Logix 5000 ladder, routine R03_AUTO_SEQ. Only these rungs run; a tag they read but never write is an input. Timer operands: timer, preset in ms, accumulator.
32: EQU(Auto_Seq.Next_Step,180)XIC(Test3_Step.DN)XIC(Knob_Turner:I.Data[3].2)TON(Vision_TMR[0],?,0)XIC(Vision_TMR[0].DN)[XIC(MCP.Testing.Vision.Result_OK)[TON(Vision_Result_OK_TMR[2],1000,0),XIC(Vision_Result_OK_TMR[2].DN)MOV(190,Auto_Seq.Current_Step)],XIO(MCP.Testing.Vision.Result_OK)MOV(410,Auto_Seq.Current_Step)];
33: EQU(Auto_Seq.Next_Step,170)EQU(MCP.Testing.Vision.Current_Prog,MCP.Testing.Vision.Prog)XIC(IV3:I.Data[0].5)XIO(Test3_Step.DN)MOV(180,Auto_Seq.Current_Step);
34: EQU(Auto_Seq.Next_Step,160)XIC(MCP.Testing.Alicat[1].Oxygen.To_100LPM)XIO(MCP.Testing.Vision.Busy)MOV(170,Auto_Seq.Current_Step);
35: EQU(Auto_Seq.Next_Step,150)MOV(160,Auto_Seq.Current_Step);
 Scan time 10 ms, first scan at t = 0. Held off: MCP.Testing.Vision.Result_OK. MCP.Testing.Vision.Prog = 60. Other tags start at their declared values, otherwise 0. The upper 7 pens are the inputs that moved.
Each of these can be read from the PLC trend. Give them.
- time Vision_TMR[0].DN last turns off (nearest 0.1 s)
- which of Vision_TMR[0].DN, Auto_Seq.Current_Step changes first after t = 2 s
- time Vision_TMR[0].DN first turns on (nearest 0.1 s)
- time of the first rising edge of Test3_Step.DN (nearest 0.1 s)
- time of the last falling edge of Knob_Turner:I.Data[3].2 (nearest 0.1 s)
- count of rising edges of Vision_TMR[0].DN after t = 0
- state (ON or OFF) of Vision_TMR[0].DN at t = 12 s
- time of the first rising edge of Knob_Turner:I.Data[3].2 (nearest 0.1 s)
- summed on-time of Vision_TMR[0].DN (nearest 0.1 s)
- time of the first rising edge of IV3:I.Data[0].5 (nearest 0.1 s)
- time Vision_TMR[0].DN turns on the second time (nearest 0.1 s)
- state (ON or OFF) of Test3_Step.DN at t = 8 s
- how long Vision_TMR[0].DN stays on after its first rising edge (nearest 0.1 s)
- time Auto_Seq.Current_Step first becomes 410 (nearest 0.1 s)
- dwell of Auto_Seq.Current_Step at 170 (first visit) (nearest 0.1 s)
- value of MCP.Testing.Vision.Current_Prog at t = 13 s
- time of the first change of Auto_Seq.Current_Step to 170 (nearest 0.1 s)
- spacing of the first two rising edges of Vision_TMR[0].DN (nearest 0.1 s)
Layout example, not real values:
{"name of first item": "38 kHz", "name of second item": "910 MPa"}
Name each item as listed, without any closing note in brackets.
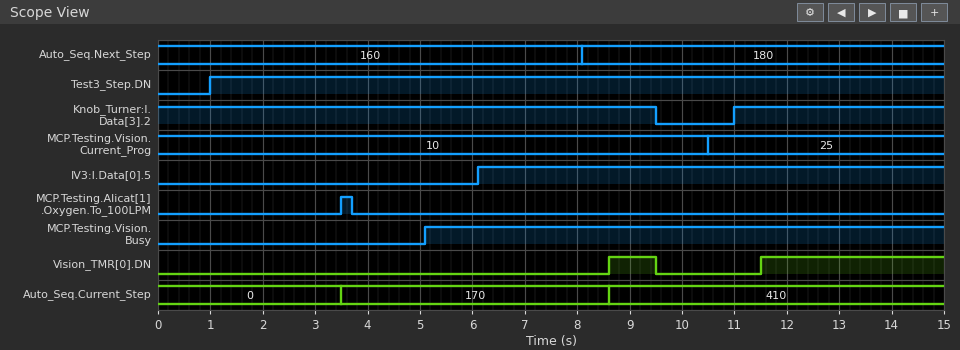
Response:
{"time Vision_TMR[0].DN last turns off": "9.5 s", "which of Vision_TMR[0].DN, Auto_Seq.Current_Step changes first after t = 2 s": "Auto_Seq.Current_Step", "time Vision_TMR[0].DN first turns on": "8.6 s", "time of the first rising edge of Test3_Step.DN": "1.0 s", "time of the last falling edge of Knob_Turner:I.Data[3].2": "9.5 s", "count of rising edges of Vision_TMR[0].DN after t = 0": "2", "state (ON or OFF) of Vision_TMR[0].DN at t = 12 s": "ON", "time of the first rising edge of Knob_Turner:I.Data[3].2": "11.0 s", "summed on-time of Vision_TMR[0].DN": "4.4 s", "time of the first rising edge of IV3:I.Data[0].5": "6.1 s", "time Vision_TMR[0].DN turns on the second time": "11.5 s", "state (ON or OFF) of Test3_Step.DN at t = 8 s": "ON", "how long Vision_TMR[0].DN stays on after its first rising edge": "0.9 s", "time Auto_Seq.Current_Step first becomes 410": "8.6 s", "dwell of Auto_Seq.Current_Step at 170 (first visit)": "5.1 s", "value of MCP.Testing.Vision.Current_Prog at t = 13 s": "25", "time of the first change of Auto_Seq.Current_Step to 170": "3.5 s", "spacing of the first two rising edges of Vision_TMR[0].DN": "2.9 s"}
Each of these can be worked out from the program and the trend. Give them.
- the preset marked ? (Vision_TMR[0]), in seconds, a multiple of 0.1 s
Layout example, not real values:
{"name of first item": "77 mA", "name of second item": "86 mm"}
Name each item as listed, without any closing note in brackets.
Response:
{"the preset marked ? (Vision_TMR[0]), in seconds, a multiple of 0.1 s": "0.5 s"}
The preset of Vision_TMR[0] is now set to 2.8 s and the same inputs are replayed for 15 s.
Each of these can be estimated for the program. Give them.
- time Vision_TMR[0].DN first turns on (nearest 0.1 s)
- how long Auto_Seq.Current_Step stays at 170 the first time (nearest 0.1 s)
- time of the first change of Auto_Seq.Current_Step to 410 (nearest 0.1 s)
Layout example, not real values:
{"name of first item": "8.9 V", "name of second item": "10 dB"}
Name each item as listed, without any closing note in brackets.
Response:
{"time Vision_TMR[0].DN first turns on": "13.8 s", "how long Auto_Seq.Current_Step stays at 170 the first time": "10.3 s", "time of the first change of Auto_Seq.Current_Step to 410": "13.8 s"}
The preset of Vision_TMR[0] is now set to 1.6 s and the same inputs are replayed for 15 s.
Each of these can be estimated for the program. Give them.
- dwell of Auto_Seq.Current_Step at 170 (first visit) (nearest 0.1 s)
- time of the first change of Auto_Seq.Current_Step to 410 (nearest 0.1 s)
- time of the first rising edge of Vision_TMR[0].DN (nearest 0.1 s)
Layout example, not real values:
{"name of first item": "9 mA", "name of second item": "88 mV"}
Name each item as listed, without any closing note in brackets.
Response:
{"dwell of Auto_Seq.Current_Step at 170 (first visit)": "9.1 s", "time of the first change of Auto_Seq.Current_Step to 410": "12.6 s", "time of the first rising edge of Vision_TMR[0].DN": "12.6 s"}
